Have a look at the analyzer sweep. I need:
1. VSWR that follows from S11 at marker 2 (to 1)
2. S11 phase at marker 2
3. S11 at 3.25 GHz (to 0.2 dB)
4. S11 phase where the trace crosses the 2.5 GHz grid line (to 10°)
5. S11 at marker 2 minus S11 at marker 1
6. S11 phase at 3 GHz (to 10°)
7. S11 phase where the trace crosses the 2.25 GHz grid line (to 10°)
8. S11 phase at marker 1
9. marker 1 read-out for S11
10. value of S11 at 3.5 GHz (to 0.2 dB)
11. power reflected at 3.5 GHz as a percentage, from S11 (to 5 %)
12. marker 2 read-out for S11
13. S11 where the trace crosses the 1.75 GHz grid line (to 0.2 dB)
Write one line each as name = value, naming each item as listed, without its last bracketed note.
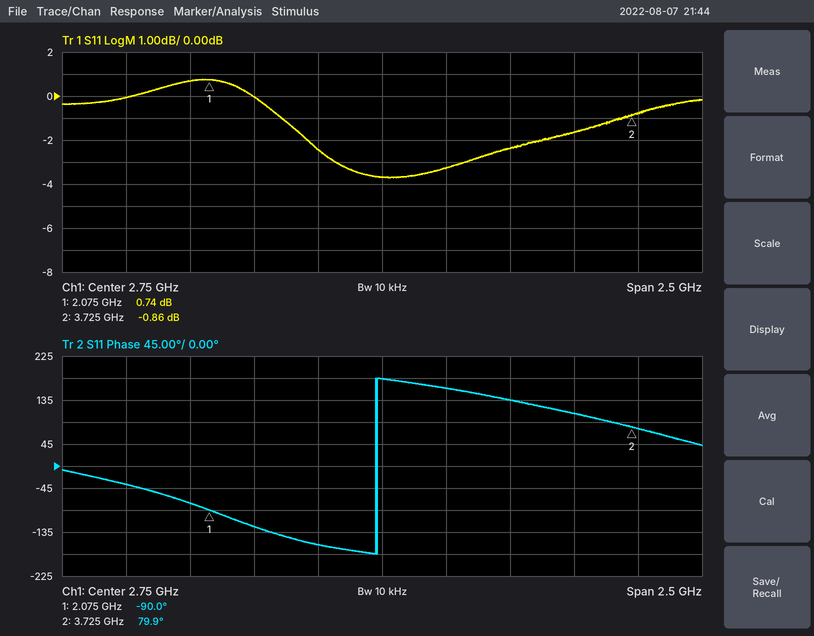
VSWR that follows from S11 at marker 2 = 20
S11 phase at marker 2 = 79.9°
S11 at 3.25 GHz = -2.4 dB
S11 phase where the trace crosses the 2.5 GHz grid line = -160°
S11 at marker 2 minus S11 at marker 1 = -1.60 dB
S11 phase at 3 GHz = 160°
S11 phase where the trace crosses the 2.25 GHz grid line = -120°
S11 phase at marker 1 = -90.0°
marker 1 read-out for S11 = 0.74 dB
value of S11 at 3.5 GHz = -1.6 dB
power reflected at 3.5 GHz as a percentage, from S11 = 70 %
marker 2 read-out for S11 = -0.86 dB
S11 where the trace crosses the 1.75 GHz grid line = 0.0 dB
